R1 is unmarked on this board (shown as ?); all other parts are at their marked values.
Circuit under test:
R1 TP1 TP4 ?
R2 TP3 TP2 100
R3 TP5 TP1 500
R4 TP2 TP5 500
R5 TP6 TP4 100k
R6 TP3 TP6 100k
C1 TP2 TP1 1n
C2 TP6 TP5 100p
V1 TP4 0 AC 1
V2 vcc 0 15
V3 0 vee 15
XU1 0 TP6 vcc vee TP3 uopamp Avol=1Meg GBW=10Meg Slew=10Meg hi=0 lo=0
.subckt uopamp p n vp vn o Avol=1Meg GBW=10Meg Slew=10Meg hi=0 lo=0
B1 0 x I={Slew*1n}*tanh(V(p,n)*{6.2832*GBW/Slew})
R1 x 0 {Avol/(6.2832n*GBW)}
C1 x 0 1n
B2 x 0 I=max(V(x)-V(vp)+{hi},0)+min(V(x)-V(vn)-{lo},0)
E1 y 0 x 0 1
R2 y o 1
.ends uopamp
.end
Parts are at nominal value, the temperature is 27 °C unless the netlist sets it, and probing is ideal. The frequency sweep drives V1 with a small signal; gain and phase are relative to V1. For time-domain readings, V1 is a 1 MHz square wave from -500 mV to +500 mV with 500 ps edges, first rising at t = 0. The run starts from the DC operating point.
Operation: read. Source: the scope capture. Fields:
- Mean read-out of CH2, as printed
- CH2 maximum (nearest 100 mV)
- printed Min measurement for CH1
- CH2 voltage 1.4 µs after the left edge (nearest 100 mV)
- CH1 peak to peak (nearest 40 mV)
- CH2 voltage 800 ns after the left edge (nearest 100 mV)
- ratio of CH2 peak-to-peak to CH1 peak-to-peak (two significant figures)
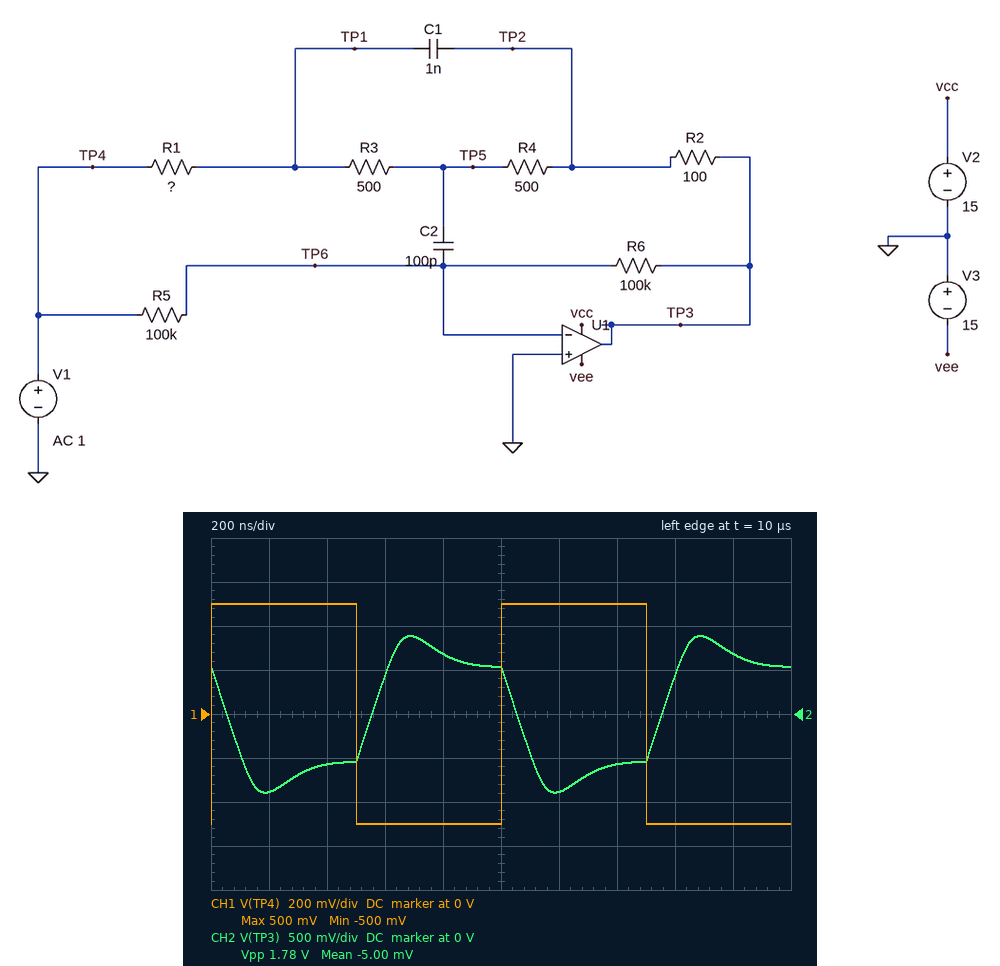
-5.00 mV
900 mV
-500 mV
-600 mV
1.00 V
700 mV
1.8
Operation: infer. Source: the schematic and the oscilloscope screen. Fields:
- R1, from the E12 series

39 Ω
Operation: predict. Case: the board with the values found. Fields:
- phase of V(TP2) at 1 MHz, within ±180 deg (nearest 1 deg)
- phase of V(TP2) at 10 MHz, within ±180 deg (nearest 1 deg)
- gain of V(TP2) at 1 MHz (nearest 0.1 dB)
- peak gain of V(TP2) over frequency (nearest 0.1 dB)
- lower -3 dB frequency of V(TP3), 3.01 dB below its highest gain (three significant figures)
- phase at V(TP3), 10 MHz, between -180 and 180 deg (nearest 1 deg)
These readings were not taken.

141 deg
23 deg
-0.4 dB
0 dB
720 kHz
108 deg
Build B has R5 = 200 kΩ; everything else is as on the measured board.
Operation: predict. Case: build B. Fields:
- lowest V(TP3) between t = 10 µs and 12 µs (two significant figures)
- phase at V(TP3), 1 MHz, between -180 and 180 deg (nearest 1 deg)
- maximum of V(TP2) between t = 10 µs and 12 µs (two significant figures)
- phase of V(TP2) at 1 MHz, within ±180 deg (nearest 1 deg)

-930 mV
-171 deg
1.1 V
142 deg
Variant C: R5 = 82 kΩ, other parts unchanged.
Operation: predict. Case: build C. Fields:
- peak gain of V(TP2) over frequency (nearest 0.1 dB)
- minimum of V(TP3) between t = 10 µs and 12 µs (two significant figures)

0.2 dB
-880 mV
